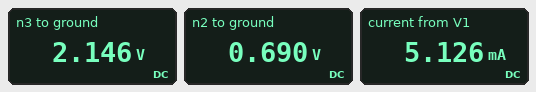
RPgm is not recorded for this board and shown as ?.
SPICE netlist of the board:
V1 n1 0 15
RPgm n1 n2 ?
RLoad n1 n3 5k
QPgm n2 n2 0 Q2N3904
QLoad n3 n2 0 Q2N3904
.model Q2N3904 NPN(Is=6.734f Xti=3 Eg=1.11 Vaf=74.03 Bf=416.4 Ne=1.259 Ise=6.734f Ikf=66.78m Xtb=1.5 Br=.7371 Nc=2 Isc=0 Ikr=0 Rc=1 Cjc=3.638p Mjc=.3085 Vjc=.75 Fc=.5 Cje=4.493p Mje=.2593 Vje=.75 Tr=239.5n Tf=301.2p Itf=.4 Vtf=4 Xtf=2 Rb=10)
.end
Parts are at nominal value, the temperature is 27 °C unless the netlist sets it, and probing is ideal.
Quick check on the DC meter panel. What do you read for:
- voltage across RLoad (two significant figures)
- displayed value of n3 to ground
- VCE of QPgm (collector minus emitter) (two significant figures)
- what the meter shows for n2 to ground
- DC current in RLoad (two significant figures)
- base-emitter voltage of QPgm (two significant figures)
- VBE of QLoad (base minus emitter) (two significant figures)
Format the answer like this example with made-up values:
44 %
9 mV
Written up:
13 V
2.146 V
690 mV
0.690 V
2.6 mA
690 mV
690 mV
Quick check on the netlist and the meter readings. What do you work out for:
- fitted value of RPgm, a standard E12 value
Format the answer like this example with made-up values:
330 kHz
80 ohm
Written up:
5.6 kΩ
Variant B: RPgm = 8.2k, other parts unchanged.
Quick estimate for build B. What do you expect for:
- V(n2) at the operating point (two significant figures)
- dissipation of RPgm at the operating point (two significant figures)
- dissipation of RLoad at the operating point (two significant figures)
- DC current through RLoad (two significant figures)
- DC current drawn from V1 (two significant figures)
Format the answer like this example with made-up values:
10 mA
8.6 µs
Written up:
680 mV
25 mW
17 mW
1.8 mA
3.6 mA
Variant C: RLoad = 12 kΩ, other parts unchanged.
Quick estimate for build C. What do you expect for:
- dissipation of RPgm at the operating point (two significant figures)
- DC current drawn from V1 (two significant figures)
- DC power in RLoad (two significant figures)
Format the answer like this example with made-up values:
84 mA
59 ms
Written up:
37 mW
3.8 mA
19 mW
